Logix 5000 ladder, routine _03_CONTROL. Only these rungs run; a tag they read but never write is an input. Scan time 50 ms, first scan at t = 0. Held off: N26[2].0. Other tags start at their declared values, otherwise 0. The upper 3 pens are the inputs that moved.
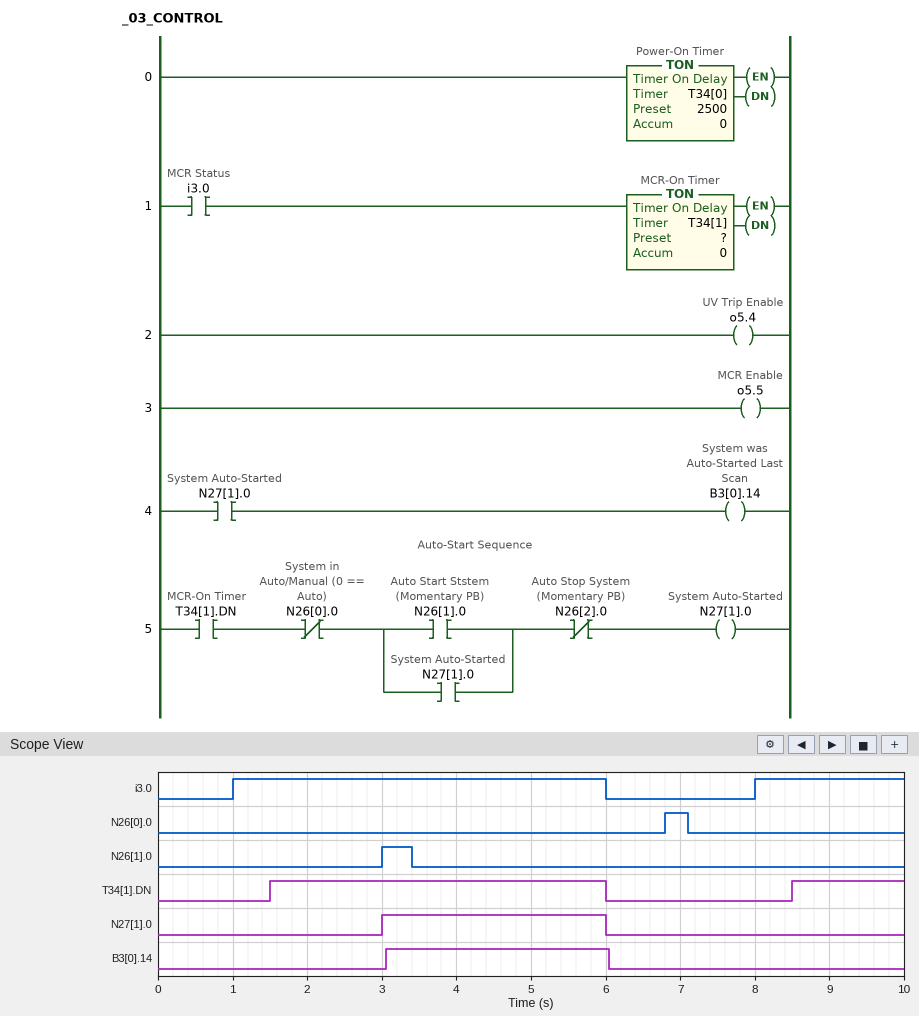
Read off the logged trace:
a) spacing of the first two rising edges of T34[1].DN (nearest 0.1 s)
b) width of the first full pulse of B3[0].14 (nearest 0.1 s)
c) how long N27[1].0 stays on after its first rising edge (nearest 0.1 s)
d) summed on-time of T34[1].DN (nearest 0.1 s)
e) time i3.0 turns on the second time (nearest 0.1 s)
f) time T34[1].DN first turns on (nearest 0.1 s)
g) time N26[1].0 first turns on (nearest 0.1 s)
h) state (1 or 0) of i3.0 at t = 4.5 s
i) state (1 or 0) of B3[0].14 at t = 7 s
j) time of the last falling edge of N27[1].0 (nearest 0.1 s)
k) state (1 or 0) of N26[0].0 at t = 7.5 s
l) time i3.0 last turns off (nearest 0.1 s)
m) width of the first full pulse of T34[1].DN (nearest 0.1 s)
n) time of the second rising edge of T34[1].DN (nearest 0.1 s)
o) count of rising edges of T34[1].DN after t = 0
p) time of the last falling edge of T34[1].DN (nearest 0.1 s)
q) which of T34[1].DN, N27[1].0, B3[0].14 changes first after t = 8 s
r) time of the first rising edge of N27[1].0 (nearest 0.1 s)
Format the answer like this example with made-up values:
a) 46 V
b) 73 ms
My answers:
a) 7.0 s
b) 3.0 s
c) 3.0 s
d) 6.0 s
e) 8.0 s
f) 1.5 s
g) 3.0 s
h) 1
i) 0
j) 6.0 s
k) 0
l) 6.0 s
m) 4.5 s
n) 8.5 s
o) 2
p) 6.0 s
q) T34[1].DN
r) 3.0 s
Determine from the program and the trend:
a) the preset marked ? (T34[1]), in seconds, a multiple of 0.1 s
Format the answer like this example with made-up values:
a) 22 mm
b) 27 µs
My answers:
a) 0.5 s
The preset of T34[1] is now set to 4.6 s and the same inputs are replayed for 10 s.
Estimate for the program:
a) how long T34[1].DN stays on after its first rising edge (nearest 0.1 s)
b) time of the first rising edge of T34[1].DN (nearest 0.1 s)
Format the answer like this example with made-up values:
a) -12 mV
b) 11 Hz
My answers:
a) 0.4 s
b) 5.6 s
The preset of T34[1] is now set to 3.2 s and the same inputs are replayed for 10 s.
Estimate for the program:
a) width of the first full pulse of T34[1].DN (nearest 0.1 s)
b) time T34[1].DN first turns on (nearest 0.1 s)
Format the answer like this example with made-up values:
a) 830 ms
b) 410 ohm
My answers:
a) 1.8 s
b) 4.2 s
